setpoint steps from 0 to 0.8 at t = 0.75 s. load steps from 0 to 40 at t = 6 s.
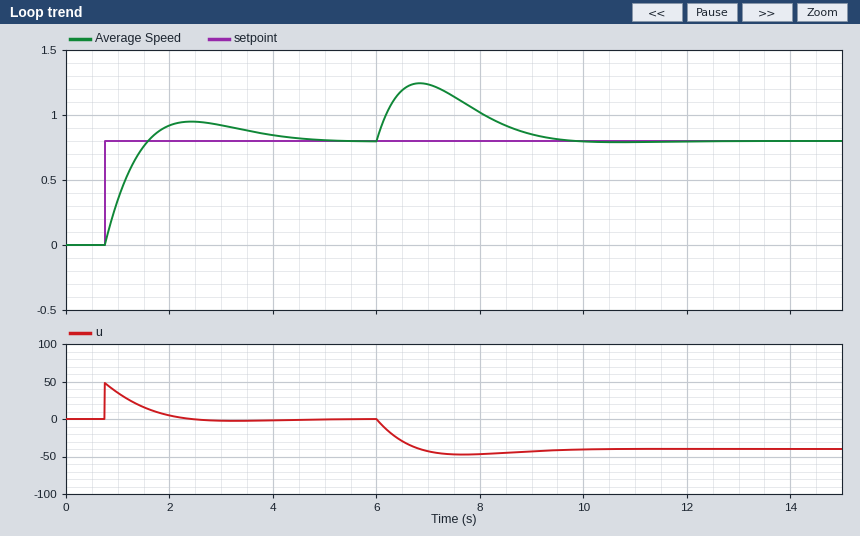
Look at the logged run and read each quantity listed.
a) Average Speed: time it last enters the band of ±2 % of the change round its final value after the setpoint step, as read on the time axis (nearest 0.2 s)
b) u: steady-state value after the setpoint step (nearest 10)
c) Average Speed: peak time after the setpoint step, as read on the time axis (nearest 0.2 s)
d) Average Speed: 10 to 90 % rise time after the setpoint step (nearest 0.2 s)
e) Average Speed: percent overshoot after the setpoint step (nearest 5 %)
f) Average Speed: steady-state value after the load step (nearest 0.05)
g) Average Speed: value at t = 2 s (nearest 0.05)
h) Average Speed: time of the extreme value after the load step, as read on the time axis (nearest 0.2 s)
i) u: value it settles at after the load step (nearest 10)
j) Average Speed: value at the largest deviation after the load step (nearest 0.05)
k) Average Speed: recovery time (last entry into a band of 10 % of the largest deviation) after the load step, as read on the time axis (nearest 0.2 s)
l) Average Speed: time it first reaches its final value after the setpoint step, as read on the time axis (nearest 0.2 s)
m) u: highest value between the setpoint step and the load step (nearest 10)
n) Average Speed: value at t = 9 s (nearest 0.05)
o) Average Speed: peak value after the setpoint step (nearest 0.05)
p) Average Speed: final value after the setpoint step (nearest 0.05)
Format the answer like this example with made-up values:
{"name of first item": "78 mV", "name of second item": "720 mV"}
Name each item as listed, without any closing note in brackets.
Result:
{"Average Speed: time it last enters the band of ±2 % of the change round its final value after the setpoint step, as read on the time axis": "4.6 s", "u: steady-state value after the setpoint step": "0", "Average Speed: peak time after the setpoint step, as read on the time axis": "2.4 s", "Average Speed: 10 to 90 % rise time after the setpoint step": "0.6 s", "Average Speed: percent overshoot after the setpoint step": "20 %", "Average Speed: steady-state value after the load step": "0.80", "Average Speed: value at t = 2 s": "0.90", "Average Speed: time of the extreme value after the load step, as read on the time axis": "6.8 s", "u: value it settles at after the load step": "-40", "Average Speed: value at the largest deviation after the load step": "1.25", "Average Speed: recovery time (last entry into a band of 10 % of the largest deviation) after the load step, as read on the time axis": "9.0 s", "Average Speed: time it first reaches its final value after the setpoint step, as read on the time axis": "1.6 s", "u: highest value between the setpoint step and the load step": "50", "Average Speed: value at t = 9 s": "0.85", "Average Speed: peak value after the setpoint step": "0.95", "Average Speed: final value after the setpoint step": "0.80"}
